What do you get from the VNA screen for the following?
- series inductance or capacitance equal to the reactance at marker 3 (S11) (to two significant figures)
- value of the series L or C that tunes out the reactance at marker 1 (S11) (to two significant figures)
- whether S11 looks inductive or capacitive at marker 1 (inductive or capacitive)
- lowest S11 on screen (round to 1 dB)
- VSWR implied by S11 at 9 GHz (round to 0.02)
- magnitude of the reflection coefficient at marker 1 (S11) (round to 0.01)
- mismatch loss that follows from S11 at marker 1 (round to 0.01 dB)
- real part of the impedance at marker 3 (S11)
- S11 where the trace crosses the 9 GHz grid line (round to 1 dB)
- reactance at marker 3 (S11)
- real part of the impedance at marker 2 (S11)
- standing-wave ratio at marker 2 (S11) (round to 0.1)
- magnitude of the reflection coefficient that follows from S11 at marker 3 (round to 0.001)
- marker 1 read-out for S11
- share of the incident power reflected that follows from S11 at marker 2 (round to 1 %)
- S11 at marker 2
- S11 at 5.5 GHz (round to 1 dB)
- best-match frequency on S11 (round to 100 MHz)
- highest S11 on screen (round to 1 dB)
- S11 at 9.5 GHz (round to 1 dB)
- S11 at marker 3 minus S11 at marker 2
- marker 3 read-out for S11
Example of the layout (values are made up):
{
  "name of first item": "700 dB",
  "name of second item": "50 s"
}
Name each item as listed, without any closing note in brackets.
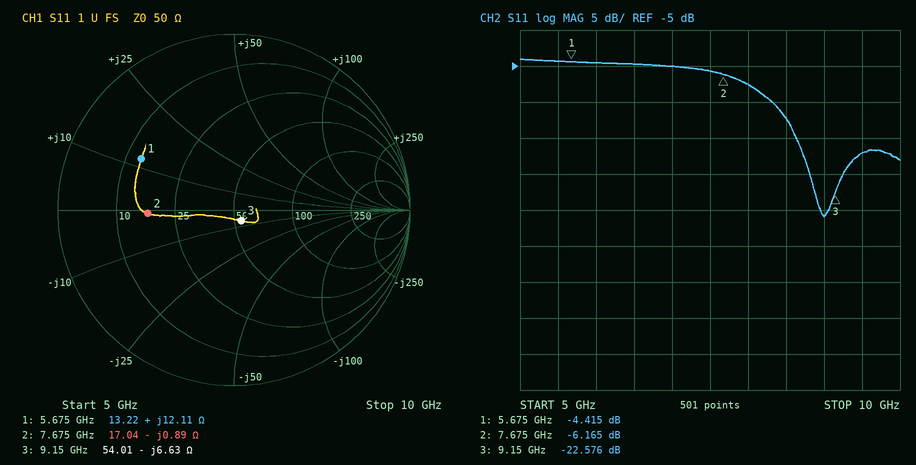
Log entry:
{
  "series inductance or capacitance equal to the reactance at marker 3 (S11)": "2.6 pF",
  "value of the series L or C that tunes out the reactance at marker 1 (S11)": "2.3 pF",
  "whether S11 looks inductive or capacitive at marker 1": "inductive",
  "lowest S11 on screen": "-26 dB",
  "VSWR implied by S11 at 9 GHz": "1.10",
  "magnitude of the reflection coefficient at marker 1 (S11)": "0.60",
  "mismatch loss that follows from S11 at marker 1": "1.95 dB",
  "real part of the impedance at marker 3": "54.01 Ω",
  "S11 where the trace crosses the 9 GHz grid line": "-26 dB",
  "reactance at marker 3": "-6.63 Ω",
  "real part of the impedance at marker 2": "17.04 Ω",
  "standing-wave ratio at marker 2 (S11)": "2.9",
  "magnitude of the reflection coefficient that follows from S11 at marker 3": "0.074",
  "marker 1 read-out for S11": "-4.415 dB",
  "share of the incident power reflected that follows from S11 at marker 2": "24 %",
  "S11 at marker 2": "-6.165 dB",
  "S11 at 5.5 GHz": "-4 dB",
  "best-match frequency on S11": "9.0 GHz",
  "highest S11 on screen": "-4 dB",
  "S11 at 9.5 GHz": "-17 dB",
  "S11 at marker 3 minus S11 at marker 2": "-16.411 dB",
  "marker 3 read-out for S11": "-22.576 dB"
}
